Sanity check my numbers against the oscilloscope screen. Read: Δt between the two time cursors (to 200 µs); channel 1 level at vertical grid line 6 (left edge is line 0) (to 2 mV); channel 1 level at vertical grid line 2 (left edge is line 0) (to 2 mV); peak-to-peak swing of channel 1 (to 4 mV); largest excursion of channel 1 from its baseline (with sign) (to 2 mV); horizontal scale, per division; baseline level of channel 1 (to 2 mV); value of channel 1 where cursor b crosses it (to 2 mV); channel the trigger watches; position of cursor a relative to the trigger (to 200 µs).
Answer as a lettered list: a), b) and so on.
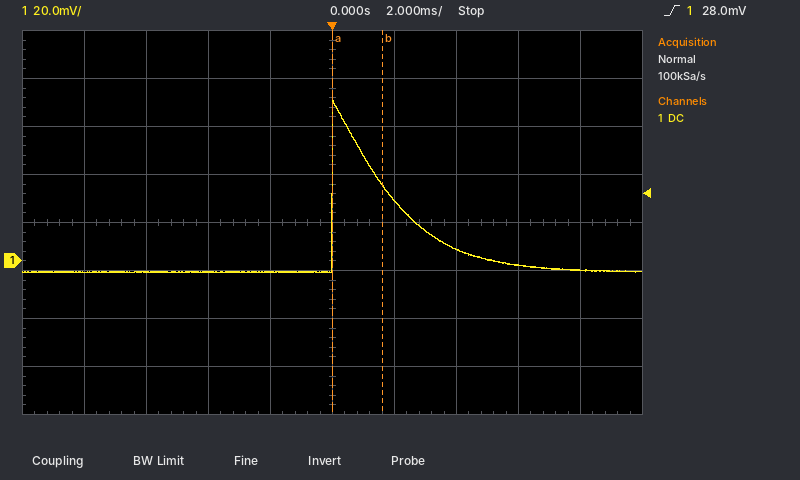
a) 1.6 ms
b) 26 mV
c) -4 mV
d) 72 mV
e) +72 mV
f) 2 ms
g) -4 mV
h) 32 mV
i) channel 1
j) 0.0 ms
